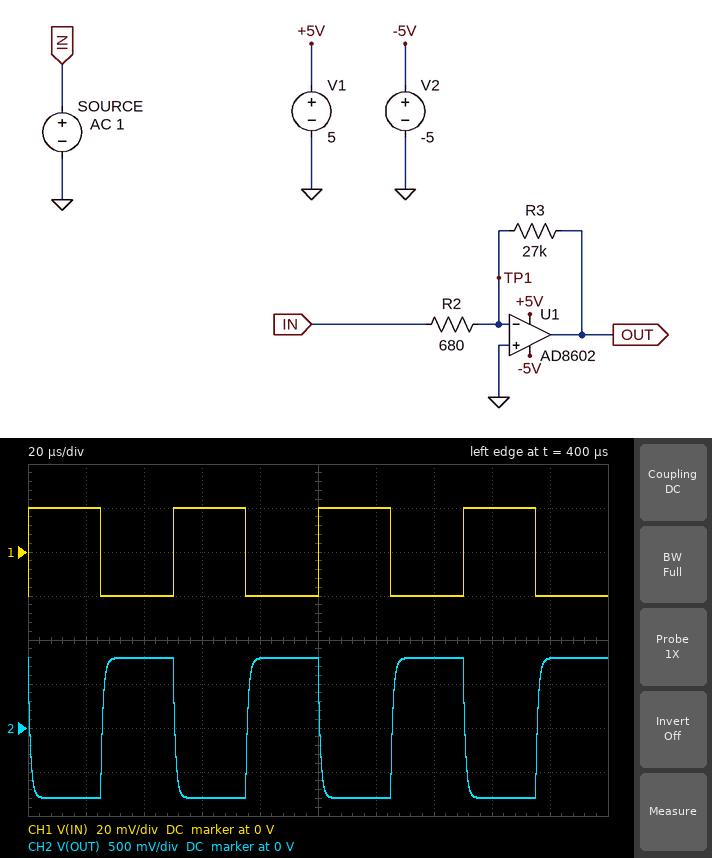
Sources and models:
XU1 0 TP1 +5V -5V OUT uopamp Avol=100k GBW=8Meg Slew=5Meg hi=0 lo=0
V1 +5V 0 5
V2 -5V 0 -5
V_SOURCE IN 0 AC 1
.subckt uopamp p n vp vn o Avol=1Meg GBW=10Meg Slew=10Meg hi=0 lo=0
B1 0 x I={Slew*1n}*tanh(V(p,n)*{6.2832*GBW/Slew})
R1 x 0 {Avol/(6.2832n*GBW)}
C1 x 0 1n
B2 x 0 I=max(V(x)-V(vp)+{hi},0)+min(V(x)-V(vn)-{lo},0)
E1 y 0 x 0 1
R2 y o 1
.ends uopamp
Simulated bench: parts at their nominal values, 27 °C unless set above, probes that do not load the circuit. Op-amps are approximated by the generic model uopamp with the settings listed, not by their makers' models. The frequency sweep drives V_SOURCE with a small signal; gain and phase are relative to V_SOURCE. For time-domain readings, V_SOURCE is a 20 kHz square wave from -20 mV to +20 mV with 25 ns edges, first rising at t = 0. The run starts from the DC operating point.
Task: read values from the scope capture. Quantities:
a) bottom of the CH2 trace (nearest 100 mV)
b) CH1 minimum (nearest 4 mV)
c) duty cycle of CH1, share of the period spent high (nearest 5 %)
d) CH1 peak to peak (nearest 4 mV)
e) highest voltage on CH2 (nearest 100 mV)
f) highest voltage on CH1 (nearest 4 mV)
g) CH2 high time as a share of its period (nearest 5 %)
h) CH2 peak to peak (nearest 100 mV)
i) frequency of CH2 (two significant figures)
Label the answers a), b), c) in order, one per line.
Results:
a) -800 mV
b) -20 mV
c) 50 %
d) 40 mV
e) 800 mV
f) 20 mV
g) 50 %
h) 1.6 V
i) 20 kHz
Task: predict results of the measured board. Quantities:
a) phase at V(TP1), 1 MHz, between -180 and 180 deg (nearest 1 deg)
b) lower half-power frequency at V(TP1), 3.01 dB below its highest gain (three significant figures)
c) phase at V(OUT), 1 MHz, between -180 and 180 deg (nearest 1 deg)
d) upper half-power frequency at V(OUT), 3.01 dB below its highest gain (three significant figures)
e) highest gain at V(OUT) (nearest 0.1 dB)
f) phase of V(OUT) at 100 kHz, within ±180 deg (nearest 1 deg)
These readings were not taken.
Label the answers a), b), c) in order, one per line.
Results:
a) 11 deg
b) 197 kHz
c) 101 deg
d) 197 kHz
e) 32.0 dB
f) 153 deg
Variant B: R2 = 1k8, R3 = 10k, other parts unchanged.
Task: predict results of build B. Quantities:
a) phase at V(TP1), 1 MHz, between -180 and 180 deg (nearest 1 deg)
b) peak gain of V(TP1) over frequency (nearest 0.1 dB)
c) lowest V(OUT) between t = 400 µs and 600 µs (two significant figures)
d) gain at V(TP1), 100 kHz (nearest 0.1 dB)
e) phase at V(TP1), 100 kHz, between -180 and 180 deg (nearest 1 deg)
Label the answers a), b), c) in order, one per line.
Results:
a) 51 deg
b) -1.4 dB
c) -110 mV
d) -23.2 dB
e) 85 deg
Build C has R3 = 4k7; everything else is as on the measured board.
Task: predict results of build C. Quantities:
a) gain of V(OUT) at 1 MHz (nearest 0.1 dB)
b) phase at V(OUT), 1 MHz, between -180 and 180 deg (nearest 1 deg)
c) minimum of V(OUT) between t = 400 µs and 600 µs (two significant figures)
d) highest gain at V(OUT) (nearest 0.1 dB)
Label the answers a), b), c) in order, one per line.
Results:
a) 13.8 dB
b) 135 deg
c) -140 mV
d) 16.8 dB
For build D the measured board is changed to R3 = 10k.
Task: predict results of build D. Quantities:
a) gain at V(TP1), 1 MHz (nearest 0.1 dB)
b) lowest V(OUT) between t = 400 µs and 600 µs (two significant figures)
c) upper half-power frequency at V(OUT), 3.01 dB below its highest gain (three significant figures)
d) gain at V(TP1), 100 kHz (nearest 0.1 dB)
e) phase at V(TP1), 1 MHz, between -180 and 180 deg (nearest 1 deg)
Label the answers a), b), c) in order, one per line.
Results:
a) -1.6 dB
b) -290 mV
c) 509 kHz
d) -14.9 dB
e) 27 deg
